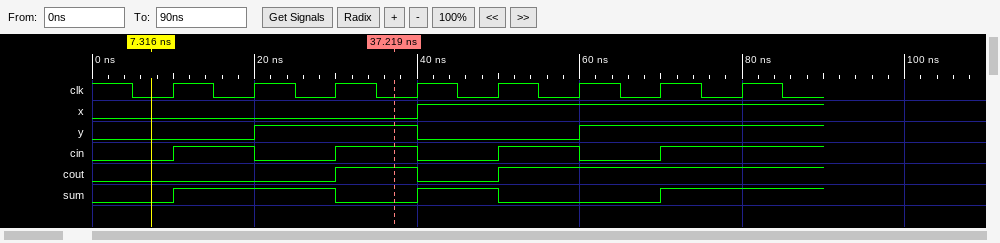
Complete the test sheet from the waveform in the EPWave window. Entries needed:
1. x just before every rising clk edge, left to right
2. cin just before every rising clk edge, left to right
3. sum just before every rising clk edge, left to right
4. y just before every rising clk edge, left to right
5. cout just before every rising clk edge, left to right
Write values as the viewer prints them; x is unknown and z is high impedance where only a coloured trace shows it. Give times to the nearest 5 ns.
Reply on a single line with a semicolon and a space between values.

0 0 0 0 1 1 1 1; 0 1 0 1 0 1 0 1; 0 1 1 0 1 0 0 1; 0 0 1 1 0 0 1 1; 0 0 0 1 0 1 1 1
